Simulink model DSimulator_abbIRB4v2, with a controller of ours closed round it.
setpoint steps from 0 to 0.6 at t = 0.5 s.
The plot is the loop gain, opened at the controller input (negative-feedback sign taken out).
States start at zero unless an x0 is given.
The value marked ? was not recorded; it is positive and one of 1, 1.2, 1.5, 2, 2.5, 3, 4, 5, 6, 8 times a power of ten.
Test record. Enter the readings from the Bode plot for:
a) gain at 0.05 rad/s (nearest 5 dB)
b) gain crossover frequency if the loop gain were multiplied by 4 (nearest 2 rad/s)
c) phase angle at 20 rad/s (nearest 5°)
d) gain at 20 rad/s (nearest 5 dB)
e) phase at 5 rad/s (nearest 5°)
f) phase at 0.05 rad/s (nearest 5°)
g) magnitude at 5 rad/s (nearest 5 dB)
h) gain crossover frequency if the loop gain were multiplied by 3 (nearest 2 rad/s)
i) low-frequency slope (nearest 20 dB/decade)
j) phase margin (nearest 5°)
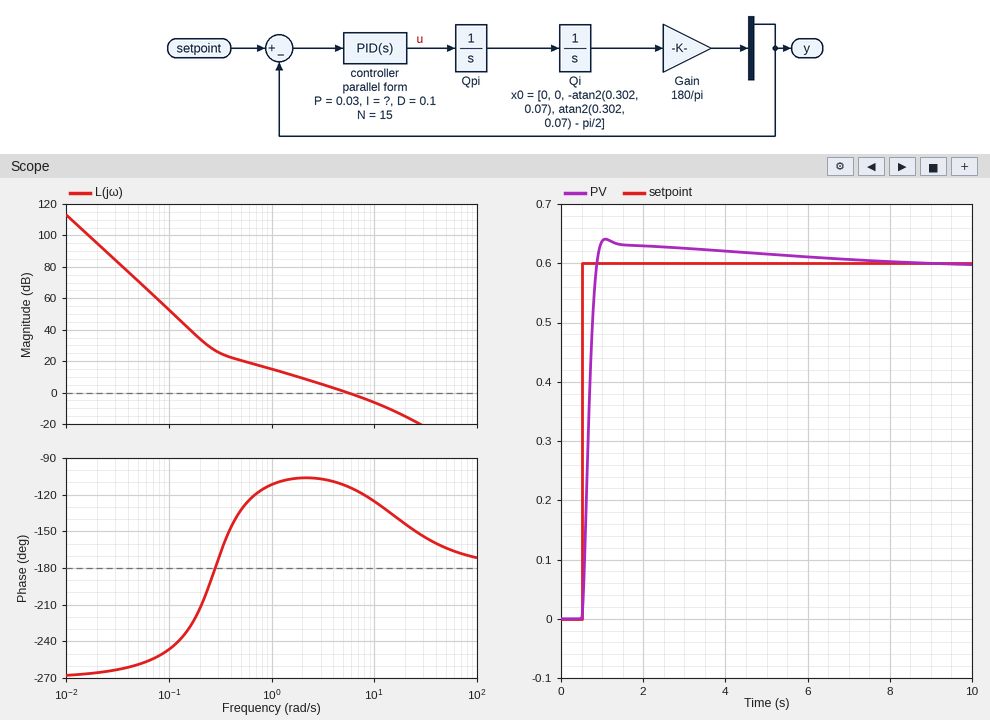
70 dB
16 rad/s
-145°
-15 dB
-110°
-260°
0 dB
14 rad/s
-60 dB/decade
65°
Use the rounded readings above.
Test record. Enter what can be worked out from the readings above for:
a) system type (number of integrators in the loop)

3
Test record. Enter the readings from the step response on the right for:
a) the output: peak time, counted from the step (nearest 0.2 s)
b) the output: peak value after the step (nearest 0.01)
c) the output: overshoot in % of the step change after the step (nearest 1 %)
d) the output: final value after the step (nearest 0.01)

0.6 s
0.64
7 %
0.60
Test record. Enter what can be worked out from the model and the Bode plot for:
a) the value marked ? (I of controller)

0.008
